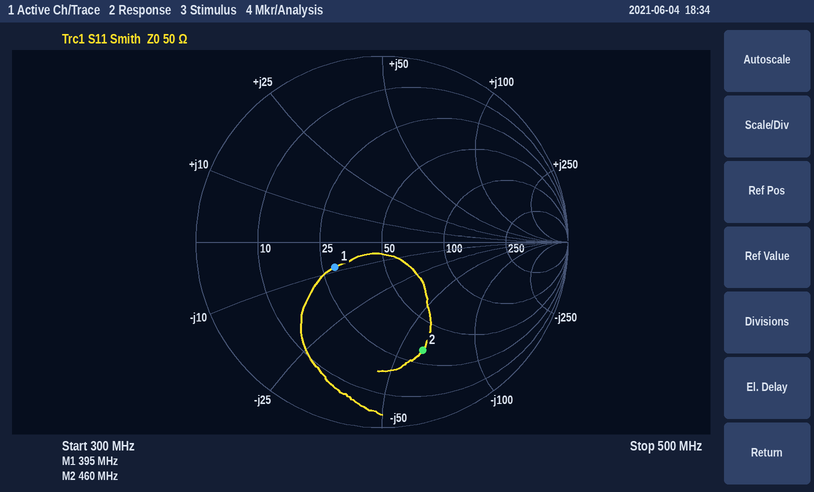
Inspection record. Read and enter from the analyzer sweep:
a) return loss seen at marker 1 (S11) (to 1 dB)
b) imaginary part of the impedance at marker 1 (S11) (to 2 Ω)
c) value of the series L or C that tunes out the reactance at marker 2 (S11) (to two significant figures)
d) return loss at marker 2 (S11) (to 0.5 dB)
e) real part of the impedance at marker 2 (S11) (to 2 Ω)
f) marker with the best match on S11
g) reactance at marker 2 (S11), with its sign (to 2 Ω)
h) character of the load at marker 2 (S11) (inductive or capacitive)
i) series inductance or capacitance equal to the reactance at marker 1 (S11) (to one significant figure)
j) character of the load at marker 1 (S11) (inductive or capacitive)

11 dB
-8 Ω
21 nH
4.0 dB
32 Ω
marker 1
-62 Ω
capacitive
50 pF
capacitive
